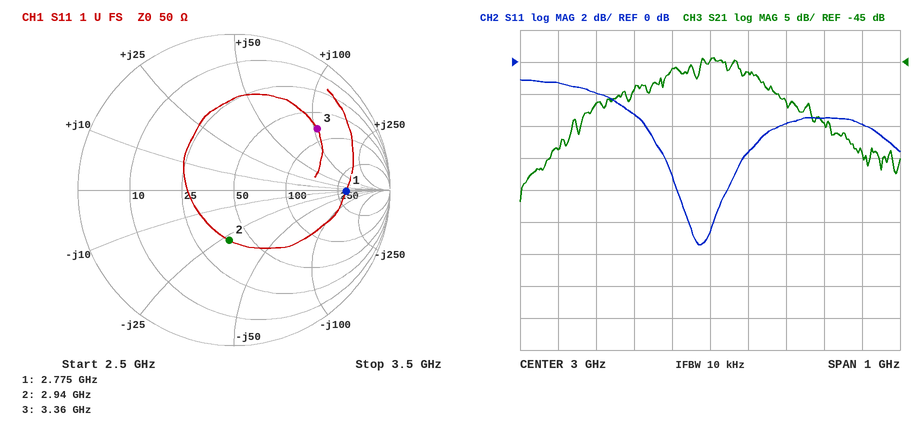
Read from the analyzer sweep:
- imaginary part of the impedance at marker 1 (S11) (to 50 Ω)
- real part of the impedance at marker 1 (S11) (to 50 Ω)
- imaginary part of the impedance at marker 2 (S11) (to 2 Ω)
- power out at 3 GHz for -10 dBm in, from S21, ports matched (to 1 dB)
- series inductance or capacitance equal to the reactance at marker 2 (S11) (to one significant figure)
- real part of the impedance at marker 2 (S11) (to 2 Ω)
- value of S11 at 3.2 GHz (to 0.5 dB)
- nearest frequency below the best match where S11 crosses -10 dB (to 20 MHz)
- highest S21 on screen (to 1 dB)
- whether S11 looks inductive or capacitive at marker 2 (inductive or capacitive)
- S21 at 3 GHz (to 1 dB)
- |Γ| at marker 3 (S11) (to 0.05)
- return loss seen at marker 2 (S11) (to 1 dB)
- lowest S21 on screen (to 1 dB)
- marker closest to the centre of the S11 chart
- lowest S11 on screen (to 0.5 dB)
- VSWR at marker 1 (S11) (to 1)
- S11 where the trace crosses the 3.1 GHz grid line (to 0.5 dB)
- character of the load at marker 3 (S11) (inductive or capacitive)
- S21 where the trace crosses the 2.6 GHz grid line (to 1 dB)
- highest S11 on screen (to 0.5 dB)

0 Ω
300 Ω
-28 Ω
-55 dBm
2 pF
38 Ω
-4.0 dB
2.94 GHz
-44 dB
capacitive
-45 dB
0.65
10 dB
-67 dB
marker 2
-11.5 dB
6
-5.5 dB
inductive
-59 dB
-1.0 dB
